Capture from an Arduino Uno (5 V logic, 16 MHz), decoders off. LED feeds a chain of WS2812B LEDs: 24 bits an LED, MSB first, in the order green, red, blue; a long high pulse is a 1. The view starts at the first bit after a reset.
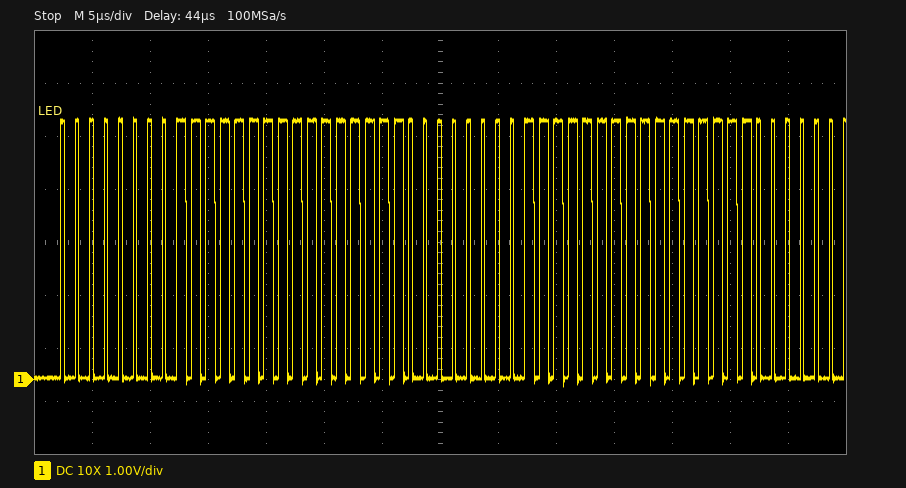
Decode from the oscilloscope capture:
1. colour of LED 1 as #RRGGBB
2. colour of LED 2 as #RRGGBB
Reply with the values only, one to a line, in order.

#FF00FF
#FF00FF
